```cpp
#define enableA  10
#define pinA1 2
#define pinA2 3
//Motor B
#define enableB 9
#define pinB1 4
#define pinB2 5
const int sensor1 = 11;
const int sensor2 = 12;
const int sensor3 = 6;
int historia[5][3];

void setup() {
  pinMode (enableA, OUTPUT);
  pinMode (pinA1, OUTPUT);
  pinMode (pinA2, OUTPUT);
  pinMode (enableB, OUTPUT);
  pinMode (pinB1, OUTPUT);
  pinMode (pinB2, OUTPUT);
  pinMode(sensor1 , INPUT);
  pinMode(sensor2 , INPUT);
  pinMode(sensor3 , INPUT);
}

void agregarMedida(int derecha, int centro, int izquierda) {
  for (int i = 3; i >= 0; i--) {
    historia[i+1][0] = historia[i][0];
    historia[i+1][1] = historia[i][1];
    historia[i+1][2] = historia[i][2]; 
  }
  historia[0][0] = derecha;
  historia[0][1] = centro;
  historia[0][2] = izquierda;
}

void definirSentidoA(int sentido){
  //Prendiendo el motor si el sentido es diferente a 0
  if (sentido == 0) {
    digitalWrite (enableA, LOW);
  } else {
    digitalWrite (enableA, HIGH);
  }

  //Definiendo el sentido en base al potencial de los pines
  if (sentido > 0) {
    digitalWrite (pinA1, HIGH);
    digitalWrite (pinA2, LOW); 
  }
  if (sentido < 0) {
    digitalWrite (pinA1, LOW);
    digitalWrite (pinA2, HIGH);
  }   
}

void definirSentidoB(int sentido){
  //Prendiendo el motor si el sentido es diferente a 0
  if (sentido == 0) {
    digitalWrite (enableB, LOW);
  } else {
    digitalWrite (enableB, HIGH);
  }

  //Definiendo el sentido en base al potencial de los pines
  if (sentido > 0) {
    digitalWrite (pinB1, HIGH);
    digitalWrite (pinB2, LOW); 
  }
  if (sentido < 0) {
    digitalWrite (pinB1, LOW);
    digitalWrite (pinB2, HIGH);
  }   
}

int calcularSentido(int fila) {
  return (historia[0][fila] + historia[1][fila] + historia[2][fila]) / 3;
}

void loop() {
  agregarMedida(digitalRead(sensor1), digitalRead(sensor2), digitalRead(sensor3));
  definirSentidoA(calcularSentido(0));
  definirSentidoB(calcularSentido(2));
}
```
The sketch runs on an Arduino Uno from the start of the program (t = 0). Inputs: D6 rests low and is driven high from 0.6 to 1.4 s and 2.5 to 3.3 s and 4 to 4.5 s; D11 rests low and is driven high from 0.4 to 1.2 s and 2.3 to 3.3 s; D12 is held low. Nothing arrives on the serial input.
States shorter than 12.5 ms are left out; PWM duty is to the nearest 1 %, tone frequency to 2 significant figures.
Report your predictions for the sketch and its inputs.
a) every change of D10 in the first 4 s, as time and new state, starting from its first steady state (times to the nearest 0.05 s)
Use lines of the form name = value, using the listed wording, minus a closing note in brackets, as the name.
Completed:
every change of D10 in the first 4 s, as time and new state, starting from its first steady state = 0 s low; 0.4 s high; 1.2 s low; 2.3 s high; 3.3 s low
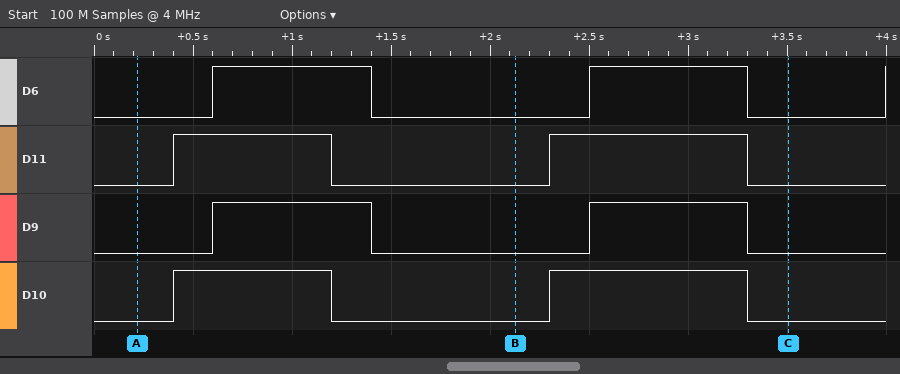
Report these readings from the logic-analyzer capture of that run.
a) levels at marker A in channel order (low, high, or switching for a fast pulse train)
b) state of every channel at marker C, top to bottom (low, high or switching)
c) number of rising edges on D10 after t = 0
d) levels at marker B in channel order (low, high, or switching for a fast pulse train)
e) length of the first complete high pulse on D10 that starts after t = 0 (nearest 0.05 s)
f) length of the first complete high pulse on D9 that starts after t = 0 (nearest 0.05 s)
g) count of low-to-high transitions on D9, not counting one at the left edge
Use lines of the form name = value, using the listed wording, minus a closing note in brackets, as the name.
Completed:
levels at marker A in channel order = D6 low, D11 low, D9 low, D10 low
state of every channel at marker C, top to bottom = D6 low, D11 low, D9 low, D10 low
number of rising edges on D10 after t = 0 = 2
levels at marker B in channel order = D6 low, D11 low, D9 low, D10 low
length of the first complete high pulse on D10 that starts after t = 0 = 0.80 s
length of the first complete high pulse on D9 that starts after t = 0 = 0.80 s
count of low-to-high transitions on D9, not counting one at the left edge = 2
